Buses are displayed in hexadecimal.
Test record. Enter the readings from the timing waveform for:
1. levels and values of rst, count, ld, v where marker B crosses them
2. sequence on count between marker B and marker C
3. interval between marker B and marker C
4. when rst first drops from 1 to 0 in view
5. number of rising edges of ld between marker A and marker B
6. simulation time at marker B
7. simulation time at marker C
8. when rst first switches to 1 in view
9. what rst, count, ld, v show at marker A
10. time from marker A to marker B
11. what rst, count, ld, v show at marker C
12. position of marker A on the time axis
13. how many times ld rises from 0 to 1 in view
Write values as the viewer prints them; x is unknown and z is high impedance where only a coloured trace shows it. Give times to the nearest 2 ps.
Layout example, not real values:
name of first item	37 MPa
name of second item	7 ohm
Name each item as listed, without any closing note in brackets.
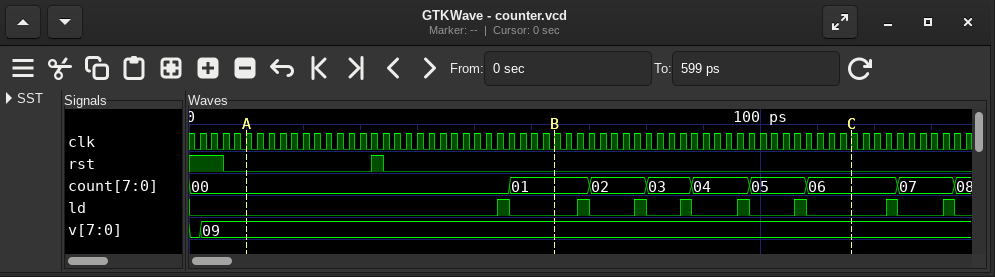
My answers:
levels and values of rst, count, ld, v where marker B crosses them	rst=0, count=01, ld=0, v=09
sequence on count between marker B and marker C	01, 02, 03, 04, 05, 06
interval between marker B and marker C	52 ps
when rst first drops from 1 to 0 in view	6 ps
number of rising edges of ld between marker A and marker B	1
simulation time at marker B	64 ps
simulation time at marker C	116 ps
when rst first switches to 1 in view	32 ps
what rst, count, ld, v show at marker A	rst=0, count=00, ld=0, v=09
time from marker A to marker B	54 ps
what rst, count, ld, v show at marker C	rst=0, count=06, ld=0, v=09
position of marker A on the time axis	10 ps
how many times ld rises from 0 to 1 in view	8
